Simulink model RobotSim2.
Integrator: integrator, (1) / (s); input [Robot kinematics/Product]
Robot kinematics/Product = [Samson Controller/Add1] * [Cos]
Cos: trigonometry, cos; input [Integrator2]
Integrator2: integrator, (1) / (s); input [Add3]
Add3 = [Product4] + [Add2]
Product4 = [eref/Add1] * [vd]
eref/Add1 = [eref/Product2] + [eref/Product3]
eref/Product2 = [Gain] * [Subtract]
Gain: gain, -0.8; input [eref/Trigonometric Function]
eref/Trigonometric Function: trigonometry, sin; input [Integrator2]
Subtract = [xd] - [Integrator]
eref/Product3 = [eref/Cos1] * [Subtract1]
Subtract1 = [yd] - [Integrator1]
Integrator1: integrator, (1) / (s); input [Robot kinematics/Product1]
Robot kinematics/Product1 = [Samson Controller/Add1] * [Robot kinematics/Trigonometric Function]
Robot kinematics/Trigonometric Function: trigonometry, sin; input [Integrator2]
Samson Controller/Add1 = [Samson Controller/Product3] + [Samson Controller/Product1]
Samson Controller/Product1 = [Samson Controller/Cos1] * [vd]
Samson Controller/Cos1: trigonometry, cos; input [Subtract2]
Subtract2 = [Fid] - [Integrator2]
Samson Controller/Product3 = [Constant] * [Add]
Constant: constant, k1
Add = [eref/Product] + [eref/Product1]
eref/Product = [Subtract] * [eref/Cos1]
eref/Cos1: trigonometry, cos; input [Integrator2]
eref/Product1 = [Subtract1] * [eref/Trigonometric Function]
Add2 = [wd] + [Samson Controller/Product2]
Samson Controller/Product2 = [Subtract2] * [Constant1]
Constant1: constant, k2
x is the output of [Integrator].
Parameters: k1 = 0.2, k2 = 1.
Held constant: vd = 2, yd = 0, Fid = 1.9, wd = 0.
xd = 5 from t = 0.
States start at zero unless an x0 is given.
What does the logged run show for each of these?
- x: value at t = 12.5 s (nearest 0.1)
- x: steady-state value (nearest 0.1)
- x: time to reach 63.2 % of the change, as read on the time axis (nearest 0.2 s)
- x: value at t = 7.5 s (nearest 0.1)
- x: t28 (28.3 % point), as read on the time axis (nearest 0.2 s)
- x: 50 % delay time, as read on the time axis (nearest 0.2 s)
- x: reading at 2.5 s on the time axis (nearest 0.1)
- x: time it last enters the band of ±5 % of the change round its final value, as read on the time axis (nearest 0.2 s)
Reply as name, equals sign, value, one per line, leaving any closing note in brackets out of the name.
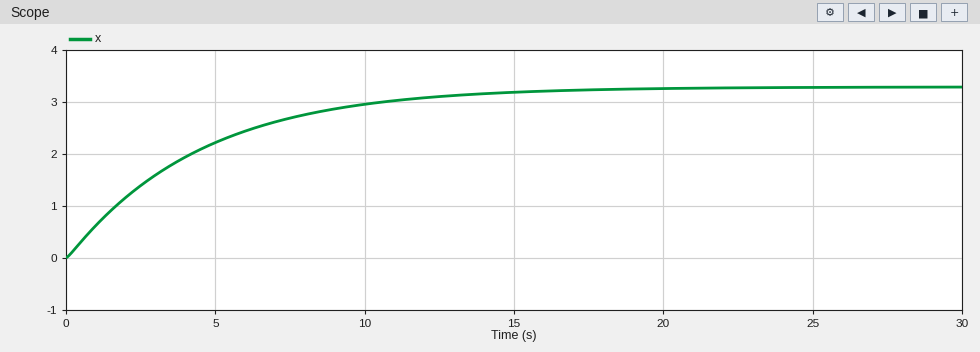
x: value at t = 12.5 s = 3.1
x: steady-state value = 3.3
x: time to reach 63.2 % of the change, as read on the time axis = 4.4 s
x: value at t = 7.5 s = 2.7
x: t28 (28.3 % point), as read on the time axis = 1.6 s
x: 50 % delay time, as read on the time axis = 3.2 s
x: reading at 2.5 s on the time axis = 1.4
x: time it last enters the band of ±5 % of the change round its final value, as read on the time axis = 13.0 s
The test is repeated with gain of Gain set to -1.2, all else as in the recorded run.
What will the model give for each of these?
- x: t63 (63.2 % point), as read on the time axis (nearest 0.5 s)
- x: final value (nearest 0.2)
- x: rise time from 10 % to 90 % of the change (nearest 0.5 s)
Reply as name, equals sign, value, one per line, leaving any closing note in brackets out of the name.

x: t63 (63.2 % point), as read on the time axis = 5.5 s
x: final value = 3.4
x: rise time from 10 % to 90 % of the change = 12.0 s
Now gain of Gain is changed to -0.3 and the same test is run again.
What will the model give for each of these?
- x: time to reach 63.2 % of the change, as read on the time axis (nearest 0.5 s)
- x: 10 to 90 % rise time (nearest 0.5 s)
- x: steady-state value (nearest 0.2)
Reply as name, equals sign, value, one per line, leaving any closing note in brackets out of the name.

x: time to reach 63.2 % of the change, as read on the time axis = 2.5 s
x: 10 to 90 % rise time = 5.5 s
x: steady-state value = 2.8
